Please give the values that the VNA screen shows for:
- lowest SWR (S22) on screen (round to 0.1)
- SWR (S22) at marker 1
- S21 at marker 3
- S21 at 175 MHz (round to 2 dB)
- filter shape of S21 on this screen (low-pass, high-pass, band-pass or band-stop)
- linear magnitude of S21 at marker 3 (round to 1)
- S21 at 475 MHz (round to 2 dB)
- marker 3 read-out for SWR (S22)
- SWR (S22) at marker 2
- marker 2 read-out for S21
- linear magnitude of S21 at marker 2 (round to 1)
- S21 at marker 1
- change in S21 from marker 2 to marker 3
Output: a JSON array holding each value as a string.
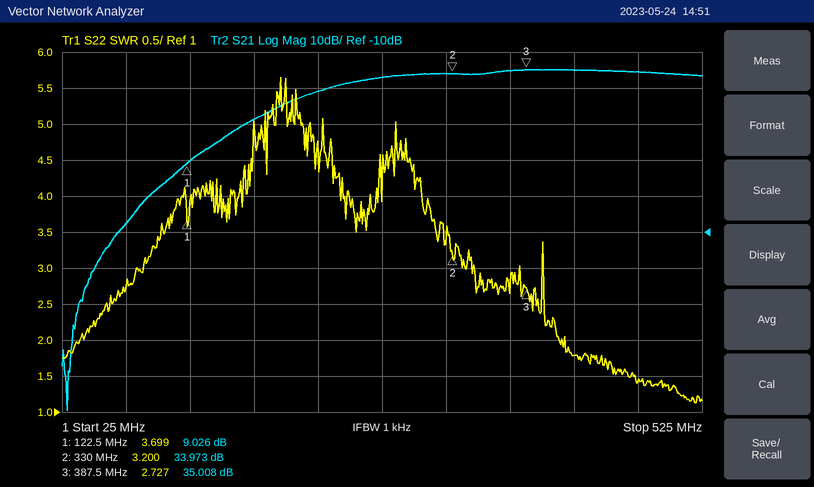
["1.1", "3.699", "35.008 dB", "22 dB", "high-pass", "56", "34 dB", "2.727", "3.200", "33.973 dB", "50", "9.026 dB", "1.035 dB"]
